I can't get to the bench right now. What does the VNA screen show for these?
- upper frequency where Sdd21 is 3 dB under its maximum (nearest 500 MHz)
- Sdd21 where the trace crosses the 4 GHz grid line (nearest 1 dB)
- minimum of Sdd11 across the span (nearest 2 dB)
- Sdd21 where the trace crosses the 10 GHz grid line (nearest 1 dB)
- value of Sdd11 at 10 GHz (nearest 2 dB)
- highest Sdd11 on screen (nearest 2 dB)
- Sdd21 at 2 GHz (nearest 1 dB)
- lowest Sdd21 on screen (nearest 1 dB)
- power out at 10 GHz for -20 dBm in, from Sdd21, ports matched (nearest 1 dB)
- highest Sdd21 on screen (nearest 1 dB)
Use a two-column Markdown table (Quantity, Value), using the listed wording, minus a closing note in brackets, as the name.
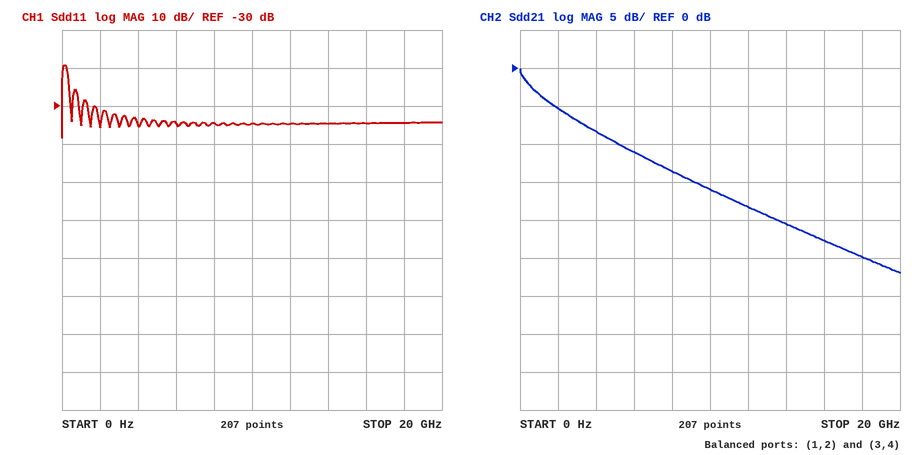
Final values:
| Quantity | Value |
|---|---|
| upper frequency where Sdd21 is 3 dB under its maximum | 1.0 GHz |
| Sdd21 where the trace crosses the 4 GHz grid line | -8 dB |
| minimum of Sdd11 across the span | -38 dB |
| Sdd21 where the trace crosses the 10 GHz grid line | -16 dB |
| value of Sdd11 at 10 GHz | -34 dB |
| highest Sdd11 on screen | -20 dB |
| Sdd21 at 2 GHz | -5 dB |
| lowest Sdd21 on screen | -27 dB |
| power out at 10 GHz for -20 dBm in, from Sdd21, ports matched | -36 dBm |
| highest Sdd21 on screen | 0 dB |
